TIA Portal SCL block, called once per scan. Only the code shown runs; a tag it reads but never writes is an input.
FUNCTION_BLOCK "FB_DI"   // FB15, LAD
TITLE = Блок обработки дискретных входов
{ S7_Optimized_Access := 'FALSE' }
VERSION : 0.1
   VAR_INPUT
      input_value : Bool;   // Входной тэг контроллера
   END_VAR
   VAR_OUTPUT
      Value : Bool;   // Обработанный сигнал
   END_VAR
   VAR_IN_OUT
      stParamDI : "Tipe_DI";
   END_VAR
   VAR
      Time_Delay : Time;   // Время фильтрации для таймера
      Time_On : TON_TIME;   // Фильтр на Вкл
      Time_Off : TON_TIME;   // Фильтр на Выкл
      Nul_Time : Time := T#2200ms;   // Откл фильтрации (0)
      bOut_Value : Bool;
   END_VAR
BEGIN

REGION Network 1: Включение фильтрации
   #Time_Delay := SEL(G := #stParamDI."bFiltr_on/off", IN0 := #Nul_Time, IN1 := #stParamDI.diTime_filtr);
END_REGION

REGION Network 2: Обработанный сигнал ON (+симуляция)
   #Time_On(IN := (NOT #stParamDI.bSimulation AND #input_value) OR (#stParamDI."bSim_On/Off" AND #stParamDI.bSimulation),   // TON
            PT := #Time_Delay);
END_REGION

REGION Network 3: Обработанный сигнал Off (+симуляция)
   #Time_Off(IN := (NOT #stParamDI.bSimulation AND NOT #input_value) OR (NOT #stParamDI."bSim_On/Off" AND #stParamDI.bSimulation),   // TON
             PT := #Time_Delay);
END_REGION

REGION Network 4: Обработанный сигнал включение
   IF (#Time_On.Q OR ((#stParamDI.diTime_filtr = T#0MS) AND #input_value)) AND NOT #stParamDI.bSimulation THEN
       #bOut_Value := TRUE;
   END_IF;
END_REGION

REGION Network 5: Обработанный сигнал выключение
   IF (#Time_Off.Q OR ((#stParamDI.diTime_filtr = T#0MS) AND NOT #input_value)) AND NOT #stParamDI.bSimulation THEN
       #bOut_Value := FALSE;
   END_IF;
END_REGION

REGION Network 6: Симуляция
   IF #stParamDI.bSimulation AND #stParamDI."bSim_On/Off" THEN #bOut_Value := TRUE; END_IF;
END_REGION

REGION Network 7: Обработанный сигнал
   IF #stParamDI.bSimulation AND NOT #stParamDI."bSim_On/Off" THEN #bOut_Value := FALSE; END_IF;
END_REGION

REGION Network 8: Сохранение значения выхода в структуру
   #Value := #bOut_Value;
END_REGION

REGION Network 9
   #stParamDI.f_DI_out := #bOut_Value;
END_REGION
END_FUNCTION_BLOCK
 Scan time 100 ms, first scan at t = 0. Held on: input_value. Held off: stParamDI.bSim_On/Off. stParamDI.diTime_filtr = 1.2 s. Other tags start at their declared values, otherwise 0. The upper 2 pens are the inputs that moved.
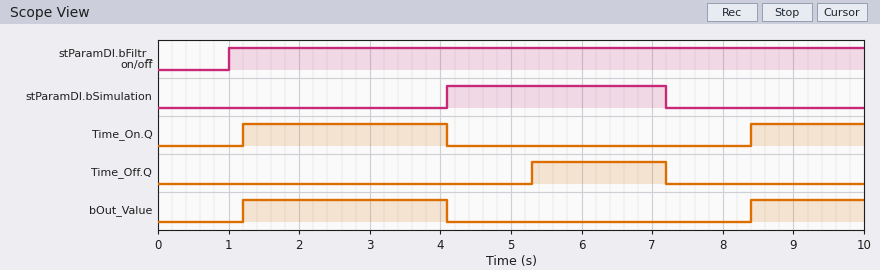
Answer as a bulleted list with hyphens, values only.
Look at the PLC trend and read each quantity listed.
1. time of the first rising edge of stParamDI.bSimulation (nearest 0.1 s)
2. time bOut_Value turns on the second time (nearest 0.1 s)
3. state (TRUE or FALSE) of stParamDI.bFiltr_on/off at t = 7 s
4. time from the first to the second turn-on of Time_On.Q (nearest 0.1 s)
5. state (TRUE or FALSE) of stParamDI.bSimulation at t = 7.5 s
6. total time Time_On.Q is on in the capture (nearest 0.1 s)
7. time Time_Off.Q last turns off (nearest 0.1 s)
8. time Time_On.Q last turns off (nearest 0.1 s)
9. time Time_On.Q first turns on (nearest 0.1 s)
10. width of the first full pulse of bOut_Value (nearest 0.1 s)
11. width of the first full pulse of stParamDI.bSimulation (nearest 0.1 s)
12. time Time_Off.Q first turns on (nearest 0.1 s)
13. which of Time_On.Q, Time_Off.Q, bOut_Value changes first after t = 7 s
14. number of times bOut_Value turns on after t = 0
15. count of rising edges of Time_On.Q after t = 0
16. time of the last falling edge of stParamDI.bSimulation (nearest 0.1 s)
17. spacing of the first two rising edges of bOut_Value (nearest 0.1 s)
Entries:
- 4.1 s
- 8.4 s
- TRUE
- 7.2 s
- FALSE
- 4.5 s
- 7.2 s
- 4.1 s
- 1.2 s
- 2.9 s
- 3.1 s
- 5.3 s
- Time_Off.Q
- 2
- 2
- 7.2 s
- 7.2 s
